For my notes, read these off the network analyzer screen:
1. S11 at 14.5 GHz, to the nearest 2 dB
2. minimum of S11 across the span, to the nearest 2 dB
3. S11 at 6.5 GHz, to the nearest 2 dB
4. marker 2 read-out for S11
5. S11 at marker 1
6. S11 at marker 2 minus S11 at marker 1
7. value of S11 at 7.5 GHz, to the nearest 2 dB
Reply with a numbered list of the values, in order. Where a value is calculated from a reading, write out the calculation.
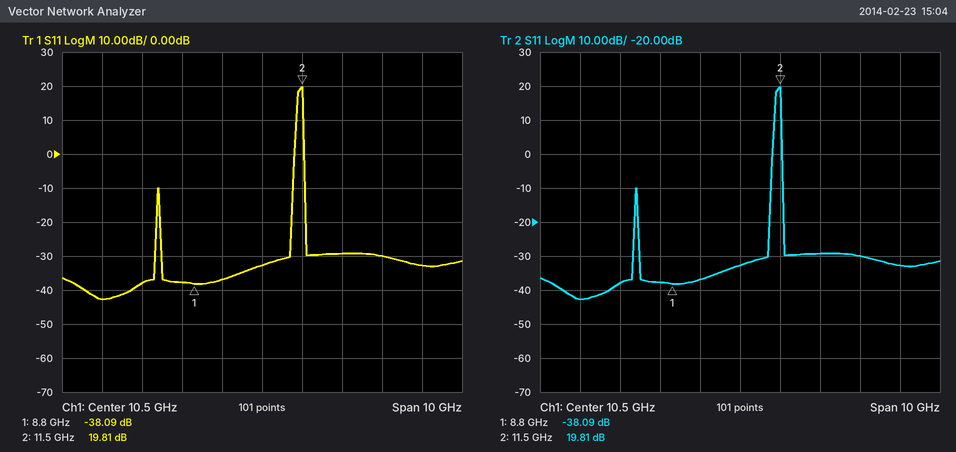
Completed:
1. -32 dB
2. -42 dB
3. -42 dB
4. 19.81 dB
5. -38.09 dB
6. 19.81 − (-38.09) = 57.90 dB
7. -38 dB
